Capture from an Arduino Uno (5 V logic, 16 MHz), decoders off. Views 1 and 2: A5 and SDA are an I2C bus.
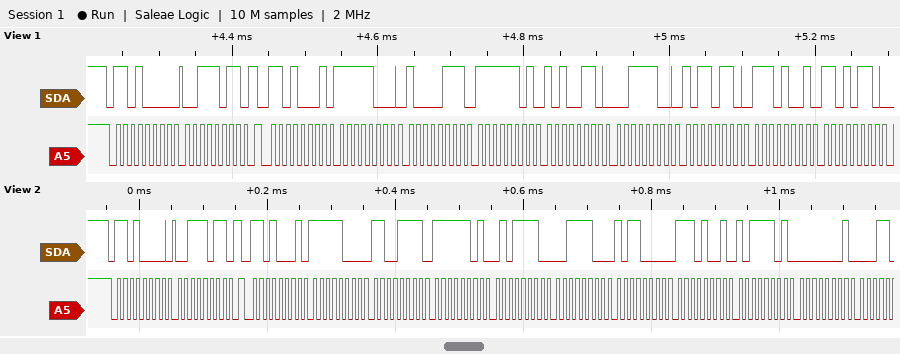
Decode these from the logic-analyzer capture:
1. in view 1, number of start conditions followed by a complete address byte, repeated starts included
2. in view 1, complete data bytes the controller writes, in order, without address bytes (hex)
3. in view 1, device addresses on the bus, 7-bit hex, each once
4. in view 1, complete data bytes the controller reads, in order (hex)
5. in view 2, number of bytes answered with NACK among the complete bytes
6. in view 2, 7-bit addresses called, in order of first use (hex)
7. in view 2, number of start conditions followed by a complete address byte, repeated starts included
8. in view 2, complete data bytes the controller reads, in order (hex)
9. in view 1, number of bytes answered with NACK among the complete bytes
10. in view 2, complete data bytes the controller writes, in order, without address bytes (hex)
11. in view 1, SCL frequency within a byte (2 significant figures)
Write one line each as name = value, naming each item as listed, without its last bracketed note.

in view 1, number of start conditions followed by a complete address byte, repeated starts included = 2
in view 1, complete data bytes the controller writes, in order, without address bytes = 3B
in view 1, device addresses on the bus, 7-bit hex, each once = 0x68
in view 1, complete data bytes the controller reads, in order = F8 87 FD A6 3C B6 E9 D6
in view 2, number of bytes answered with NACK among the complete bytes = 0
in view 2, 7-bit addresses called, in order of first use = 0x68
in view 2, number of start conditions followed by a complete address byte, repeated starts included = 2
in view 2, complete data bytes the controller reads, in order = F8 CF FD 5E 3C B0 E9 BD 01
in view 1, number of bytes answered with NACK among the complete bytes = 0
in view 2, complete data bytes the controller writes, in order, without address bytes = 3B
in view 1, SCL frequency within a byte = 100 kHz
